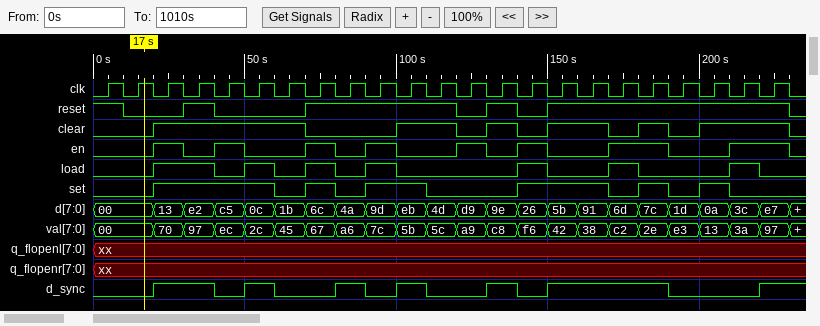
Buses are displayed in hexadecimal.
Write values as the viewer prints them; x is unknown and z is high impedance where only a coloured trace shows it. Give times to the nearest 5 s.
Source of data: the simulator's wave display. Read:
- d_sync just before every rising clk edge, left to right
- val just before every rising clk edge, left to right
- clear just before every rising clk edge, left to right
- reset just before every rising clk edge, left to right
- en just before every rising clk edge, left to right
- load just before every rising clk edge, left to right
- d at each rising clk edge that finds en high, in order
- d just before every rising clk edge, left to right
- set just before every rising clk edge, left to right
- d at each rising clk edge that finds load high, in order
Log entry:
0 0 1 1 0 1 0 0 1 0 1 0 0 1 0 1 1 1 1 0 0 0 1
00, 00, 70, 97, ec, 2c, 45, 67, a6, 7c, 5b, 5c, a9, c8, f6, 42, 38, c2, 2e, e3, 13, 3a, 97
0 0 1 1 1 1 1 0 0 0 1 1 0 1 0 1 1 0 1 0 1 1 1
1 0 0 1 0 0 0 1 1 1 1 1 0 1 0 1 1 1 1 1 1 1 1
0 0 1 0 1 0 0 1 0 1 0 0 1 0 1 0 0 1 1 0 0 1 1
0 0 1 1 0 1 0 1 0 1 0 0 0 0 1 0 0 1 0 0 0 1 0
13, c5, 6c, 9d, d9, 26, 6d, 7c, 3c, e7
00, 00, 13, e2, c5, 0c, 1b, 6c, 4a, 9d, eb, 4d, d9, 9e, 26, 5b, 91, 6d, 7c, 1d, 0a, 3c, e7
0 0 1 1 1 1 0 1 0 1 1 0 0 0 1 1 1 0 1 0 1 0 0
13, e2, 0c, 6c, 9d, 26, 6d, 3c
